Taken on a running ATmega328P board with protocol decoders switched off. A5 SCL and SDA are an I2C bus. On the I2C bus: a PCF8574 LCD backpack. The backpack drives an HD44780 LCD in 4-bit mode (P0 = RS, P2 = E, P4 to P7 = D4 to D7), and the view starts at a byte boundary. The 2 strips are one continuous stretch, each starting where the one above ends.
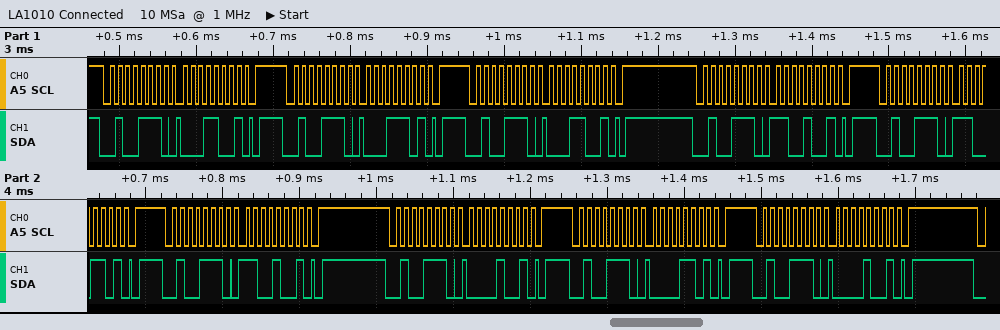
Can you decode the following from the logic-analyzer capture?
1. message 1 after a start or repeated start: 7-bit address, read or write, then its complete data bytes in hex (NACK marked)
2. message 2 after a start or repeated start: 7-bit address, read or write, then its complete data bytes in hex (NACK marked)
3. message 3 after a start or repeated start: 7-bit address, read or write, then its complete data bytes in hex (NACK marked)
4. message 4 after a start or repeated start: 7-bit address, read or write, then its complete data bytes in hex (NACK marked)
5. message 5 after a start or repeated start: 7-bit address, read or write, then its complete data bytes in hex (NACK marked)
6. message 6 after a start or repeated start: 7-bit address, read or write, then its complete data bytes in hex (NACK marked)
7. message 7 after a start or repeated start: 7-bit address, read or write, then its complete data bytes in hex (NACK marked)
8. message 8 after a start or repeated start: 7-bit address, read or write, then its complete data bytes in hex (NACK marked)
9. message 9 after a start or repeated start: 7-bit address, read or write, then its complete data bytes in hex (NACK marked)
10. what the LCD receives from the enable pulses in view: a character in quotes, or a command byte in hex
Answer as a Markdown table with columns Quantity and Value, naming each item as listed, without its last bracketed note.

| Quantity | Value |
|---|---|
| message 1 after a start or repeated start: 7-bit address, read or write, then its complete data bytes in hex | 0x27 write: 19 |
| message 2 after a start or repeated start: 7-bit address, read or write, then its complete data bytes in hex | 0x27 write: 1D |
| message 3 after a start or repeated start: 7-bit address, read or write, then its complete data bytes in hex | 0x27 write: 19 |
| message 4 after a start or repeated start: 7-bit address, read or write, then its complete data bytes in hex | 0x27 write: C9 |
| message 5 after a start or repeated start: 7-bit address, read or write, then its complete data bytes in hex | 0x27 write: CD |
| message 6 after a start or repeated start: 7-bit address, read or write, then its complete data bytes in hex | 0x27 write: C9 |
| message 7 after a start or repeated start: 7-bit address, read or write, then its complete data bytes in hex | 0x27 write: 09 |
| message 8 after a start or repeated start: 7-bit address, read or write, then its complete data bytes in hex | 0x27 write: 0D |
| message 9 after a start or repeated start: 7-bit address, read or write, then its complete data bytes in hex | 0x27 write: 09 |
| what the LCD receives from the enable pulses in view: a character in quotes, or a command byte in hex | data 0x1C |
